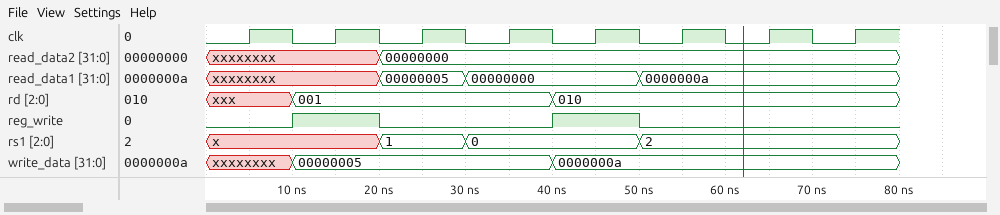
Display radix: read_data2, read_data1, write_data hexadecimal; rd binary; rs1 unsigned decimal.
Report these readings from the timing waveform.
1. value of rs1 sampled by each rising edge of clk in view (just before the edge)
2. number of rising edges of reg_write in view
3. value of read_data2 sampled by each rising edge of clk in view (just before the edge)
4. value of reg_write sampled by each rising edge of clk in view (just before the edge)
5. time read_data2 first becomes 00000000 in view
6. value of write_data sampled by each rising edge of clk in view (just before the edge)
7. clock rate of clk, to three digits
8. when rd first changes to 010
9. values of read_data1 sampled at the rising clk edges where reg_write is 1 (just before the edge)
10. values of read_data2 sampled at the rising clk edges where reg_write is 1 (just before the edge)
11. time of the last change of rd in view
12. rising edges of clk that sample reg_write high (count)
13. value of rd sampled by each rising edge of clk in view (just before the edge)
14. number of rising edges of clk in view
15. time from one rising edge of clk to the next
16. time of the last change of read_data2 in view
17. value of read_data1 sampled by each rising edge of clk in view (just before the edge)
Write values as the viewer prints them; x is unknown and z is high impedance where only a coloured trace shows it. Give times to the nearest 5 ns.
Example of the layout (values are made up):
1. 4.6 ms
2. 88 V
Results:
1. x, x, 1, 0, 0, 2, 2, 2
2. 2
3. xxxxxxxx, xxxxxxxx, 00000000, 00000000, 00000000, 00000000, 00000000, 00000000
4. 0 1 0 0 1 0 0 0
5. 20 ns
6. xxxxxxxx, 00000005, 00000005, 00000005, 0000000a, 0000000a, 0000000a, 0000000a
7. 100 MHz
8. 40 ns
9. xxxxxxxx, 00000000
10. xxxxxxxx, 00000000
11. 40 ns
12. 2
13. xxx, 001, 001, 001, 010, 010, 010, 010
14. 8
15. 10 ns
16. 20 ns
17. xxxxxxxx, xxxxxxxx, 00000005, 00000000, 00000000, 0000000a, 0000000a, 0000000a
